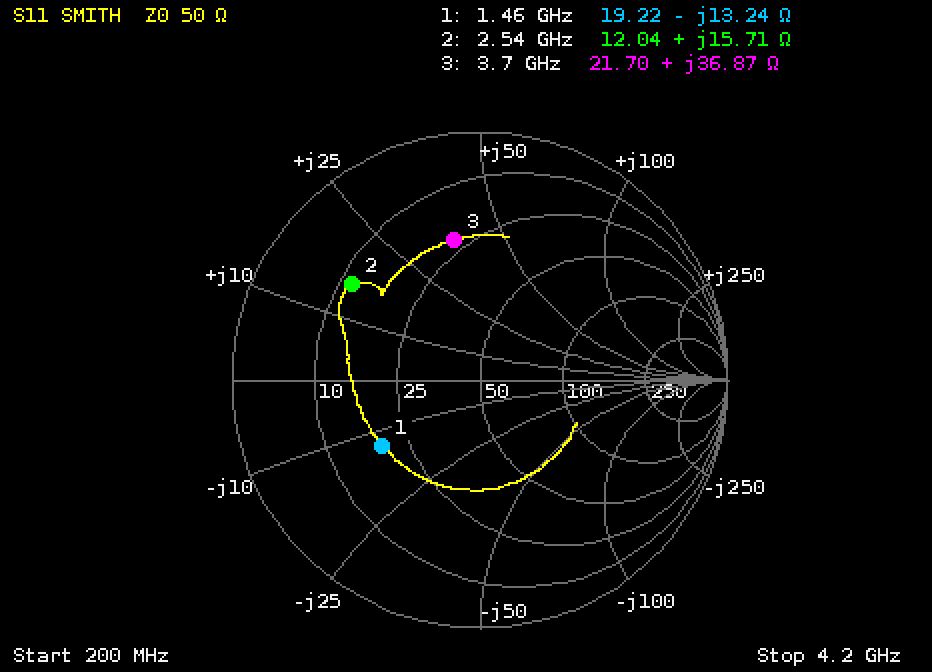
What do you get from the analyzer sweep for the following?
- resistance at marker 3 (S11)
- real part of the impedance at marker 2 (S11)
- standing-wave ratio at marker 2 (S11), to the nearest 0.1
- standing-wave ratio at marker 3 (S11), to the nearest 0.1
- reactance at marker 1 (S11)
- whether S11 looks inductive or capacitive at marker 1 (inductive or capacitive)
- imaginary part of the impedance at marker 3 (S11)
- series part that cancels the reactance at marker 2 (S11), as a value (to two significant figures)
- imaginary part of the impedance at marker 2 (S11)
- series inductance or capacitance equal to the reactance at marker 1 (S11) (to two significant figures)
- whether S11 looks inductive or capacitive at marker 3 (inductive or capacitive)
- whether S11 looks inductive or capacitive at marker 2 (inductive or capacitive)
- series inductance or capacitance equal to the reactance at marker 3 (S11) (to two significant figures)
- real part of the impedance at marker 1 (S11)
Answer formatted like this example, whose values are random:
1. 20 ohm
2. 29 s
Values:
1. 21.70 Ω
2. 12.04 Ω
3. 4.6
4. 3.7
5. -13.24 Ω
6. capacitive
7. +36.87 Ω
8. 4.0 pF
9. +15.71 Ω
10. 8.2 pF
11. inductive
12. inductive
13. 1.6 nH
14. 19.22 Ω
